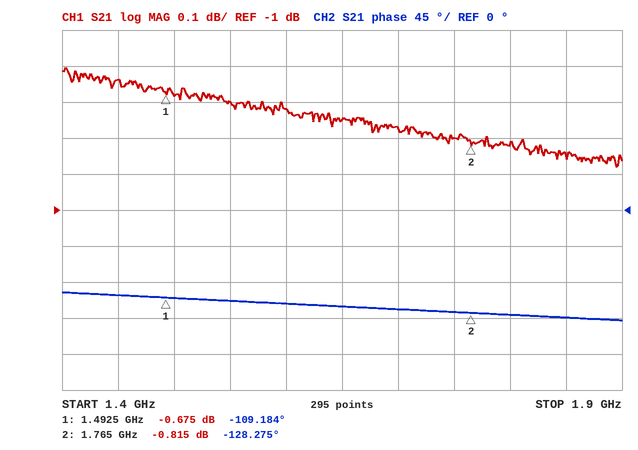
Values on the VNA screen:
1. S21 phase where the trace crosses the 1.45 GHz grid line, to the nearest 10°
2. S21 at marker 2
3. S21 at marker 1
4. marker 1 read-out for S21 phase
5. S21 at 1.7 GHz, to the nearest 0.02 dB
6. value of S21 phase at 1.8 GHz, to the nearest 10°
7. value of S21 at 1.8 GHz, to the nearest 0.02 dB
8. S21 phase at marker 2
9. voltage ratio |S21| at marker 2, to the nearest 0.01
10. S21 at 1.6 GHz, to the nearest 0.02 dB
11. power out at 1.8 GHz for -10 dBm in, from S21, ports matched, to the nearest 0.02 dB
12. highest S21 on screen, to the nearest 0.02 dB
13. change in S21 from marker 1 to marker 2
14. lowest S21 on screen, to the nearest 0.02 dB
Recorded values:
-110°
-0.815 dB
-0.675 dB
-109.184°
-0.78 dB
-130°
-0.82 dB
-128.275°
0.91
-0.72 dB
-10.82 dBm
-0.60 dB
-0.140 dB
-0.88 dB
